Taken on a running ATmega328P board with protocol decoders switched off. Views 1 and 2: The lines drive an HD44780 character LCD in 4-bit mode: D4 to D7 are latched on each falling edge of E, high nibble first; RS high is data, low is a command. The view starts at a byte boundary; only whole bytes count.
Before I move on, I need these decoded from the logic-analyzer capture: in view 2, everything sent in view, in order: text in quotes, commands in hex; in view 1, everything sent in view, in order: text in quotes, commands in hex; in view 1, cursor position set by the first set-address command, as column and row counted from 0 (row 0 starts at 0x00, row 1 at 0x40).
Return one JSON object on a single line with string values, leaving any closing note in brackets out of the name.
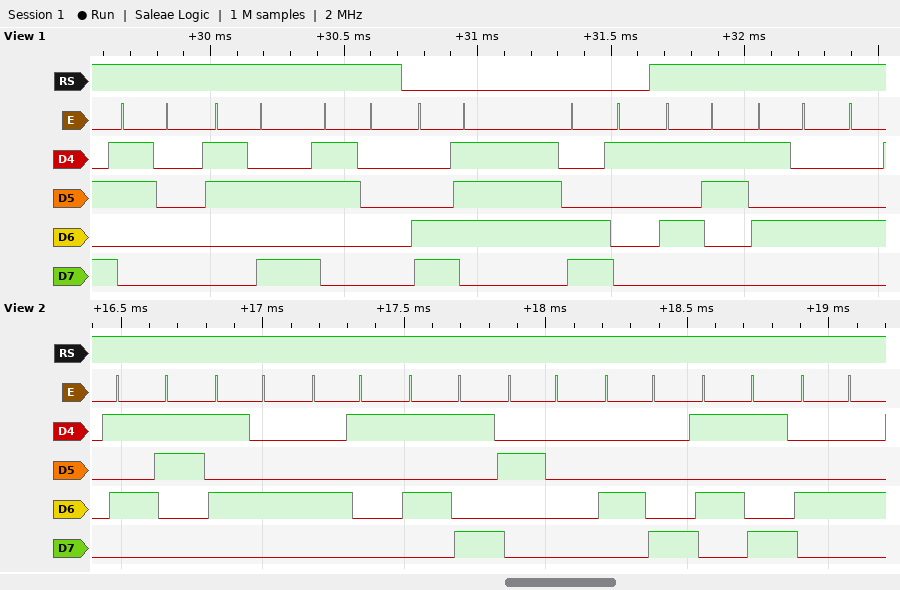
{"in view 2, everything sent in view, in order: text in quotes, commands in hex": "\"STAY HYD\"", "in view 1, everything sent in view, in order: text in quotes, commands in hex": "\"0:0\" 0xC7 0xC1 \"ST\"", "in view 1, cursor position set by the first set-address command, as column and row counted from 0": "column 7, row 1"}
